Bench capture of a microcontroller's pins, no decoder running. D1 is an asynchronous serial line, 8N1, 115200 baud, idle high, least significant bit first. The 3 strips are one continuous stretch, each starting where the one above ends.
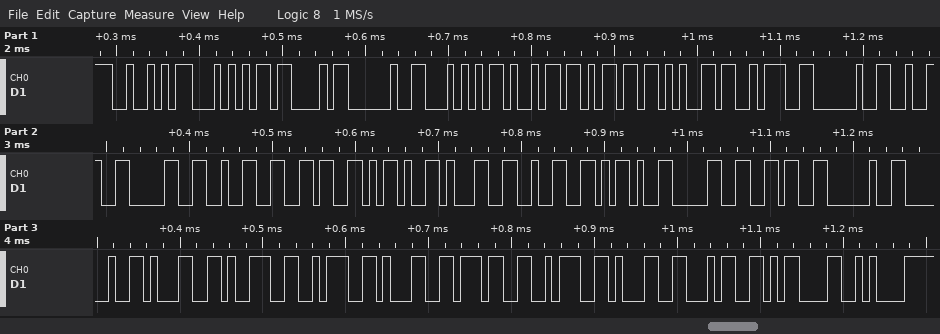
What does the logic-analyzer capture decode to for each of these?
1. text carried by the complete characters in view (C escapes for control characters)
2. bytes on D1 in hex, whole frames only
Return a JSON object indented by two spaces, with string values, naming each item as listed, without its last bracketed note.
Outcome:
{
  "text carried by the complete characters in view": "\"RTC Time: 2026-12-06  19:17:14\\r\\n\"",
  "bytes on D1 in hex, whole frames only": "52 54 43 20 54 69 6D 65 3A 20 32 30 32 36 2D 31 32 2D 30 36 20 20 31 39 3A 31 37 3A 31 34 0D 0A"
}
